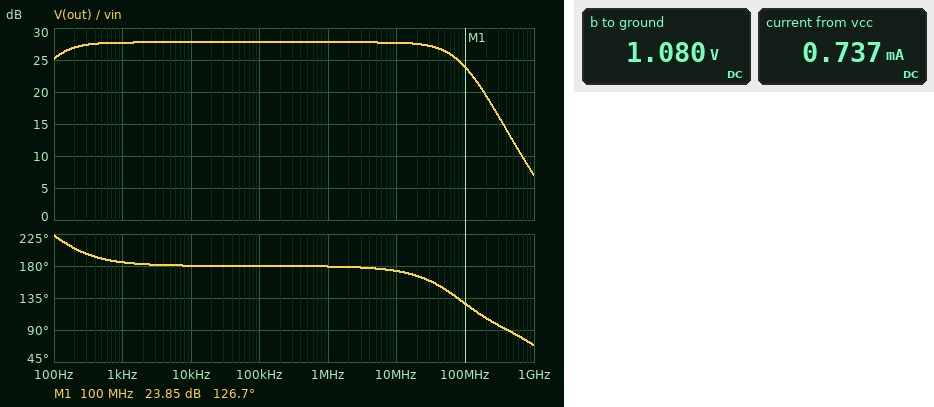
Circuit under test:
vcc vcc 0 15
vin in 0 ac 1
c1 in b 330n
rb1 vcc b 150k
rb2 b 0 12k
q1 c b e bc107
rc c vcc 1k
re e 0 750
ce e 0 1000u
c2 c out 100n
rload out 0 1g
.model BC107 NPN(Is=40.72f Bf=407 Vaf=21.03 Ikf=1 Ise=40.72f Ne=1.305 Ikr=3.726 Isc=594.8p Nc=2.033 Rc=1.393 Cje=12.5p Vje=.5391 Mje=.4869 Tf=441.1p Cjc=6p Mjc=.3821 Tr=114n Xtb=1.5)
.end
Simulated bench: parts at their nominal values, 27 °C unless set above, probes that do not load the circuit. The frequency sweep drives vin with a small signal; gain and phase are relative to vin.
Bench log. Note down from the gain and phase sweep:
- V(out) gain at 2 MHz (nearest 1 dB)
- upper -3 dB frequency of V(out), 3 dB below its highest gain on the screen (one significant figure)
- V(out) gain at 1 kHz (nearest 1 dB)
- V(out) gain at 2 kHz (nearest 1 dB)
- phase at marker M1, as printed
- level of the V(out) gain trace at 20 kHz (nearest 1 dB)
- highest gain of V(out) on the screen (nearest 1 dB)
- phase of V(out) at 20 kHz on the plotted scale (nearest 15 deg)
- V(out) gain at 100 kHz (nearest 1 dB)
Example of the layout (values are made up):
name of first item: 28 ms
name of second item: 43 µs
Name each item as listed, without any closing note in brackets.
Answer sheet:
V(out) gain at 2 MHz: 28 dB
upper -3 dB frequency of V(out), 3 dB below its highest gain on the screen: 80 MHz
V(out) gain at 1 kHz: 28 dB
V(out) gain at 2 kHz: 28 dB
phase at marker M1, as printed: 126.7 deg
level of the V(out) gain trace at 20 kHz: 28 dB
highest gain of V(out) on the screen: 28 dB
phase of V(out) at 20 kHz on the plotted scale: 180 deg
V(out) gain at 100 kHz: 28 dB
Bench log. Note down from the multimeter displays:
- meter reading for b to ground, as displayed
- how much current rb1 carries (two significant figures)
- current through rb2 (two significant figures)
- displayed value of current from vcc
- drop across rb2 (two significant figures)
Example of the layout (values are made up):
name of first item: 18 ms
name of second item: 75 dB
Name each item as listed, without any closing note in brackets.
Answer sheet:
meter reading for b to ground, as displayed: 1.080 V
how much current rb1 carries: 93 µA
current through rb2: 90 µA
displayed value of current from vcc: 0.737 mA
drop across rb2: 1.1 V
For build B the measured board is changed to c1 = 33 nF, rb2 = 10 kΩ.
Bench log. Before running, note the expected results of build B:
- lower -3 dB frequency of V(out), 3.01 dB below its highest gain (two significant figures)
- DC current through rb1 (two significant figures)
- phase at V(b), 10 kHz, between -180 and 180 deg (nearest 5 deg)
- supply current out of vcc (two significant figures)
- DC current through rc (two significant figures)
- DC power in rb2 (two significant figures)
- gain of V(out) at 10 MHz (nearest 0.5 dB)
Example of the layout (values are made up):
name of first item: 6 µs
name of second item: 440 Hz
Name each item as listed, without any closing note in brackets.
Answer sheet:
lower -3 dB frequency of V(out), 3.01 dB below its highest gain: 830 Hz
DC current through rb1: 94 µA
phase at V(b), 10 kHz, between -180 and 180 deg: 5 deg
supply current out of vcc: 540 µA
DC current through rc: 440 µA
DC power in rb2: 84 µW
gain of V(out) at 10 MHz: 24.5 dB
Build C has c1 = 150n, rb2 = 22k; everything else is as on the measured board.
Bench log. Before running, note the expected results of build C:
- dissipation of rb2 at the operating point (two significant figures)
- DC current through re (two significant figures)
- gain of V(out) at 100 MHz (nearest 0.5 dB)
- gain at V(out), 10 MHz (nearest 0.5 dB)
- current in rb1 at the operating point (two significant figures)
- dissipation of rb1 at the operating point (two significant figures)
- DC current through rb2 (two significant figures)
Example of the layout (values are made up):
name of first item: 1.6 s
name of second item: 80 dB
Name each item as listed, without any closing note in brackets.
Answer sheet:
dissipation of rb2 at the operating point: 150 µW
DC current through re: 1.6 mA
gain of V(out) at 100 MHz: 31.0 dB
gain at V(out), 10 MHz: 35.0 dB
current in rb1 at the operating point: 88 µA
dissipation of rb1 at the operating point: 1.2 mW
DC current through rb2: 82 µA
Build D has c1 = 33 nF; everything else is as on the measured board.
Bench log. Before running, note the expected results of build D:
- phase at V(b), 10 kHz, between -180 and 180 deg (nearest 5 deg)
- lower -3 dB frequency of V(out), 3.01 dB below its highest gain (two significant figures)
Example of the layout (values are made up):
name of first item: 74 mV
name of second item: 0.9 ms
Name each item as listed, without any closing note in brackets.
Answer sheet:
phase at V(b), 10 kHz, between -180 and 180 deg: 5 deg
lower -3 dB frequency of V(out), 3.01 dB below its highest gain: 880 Hz
